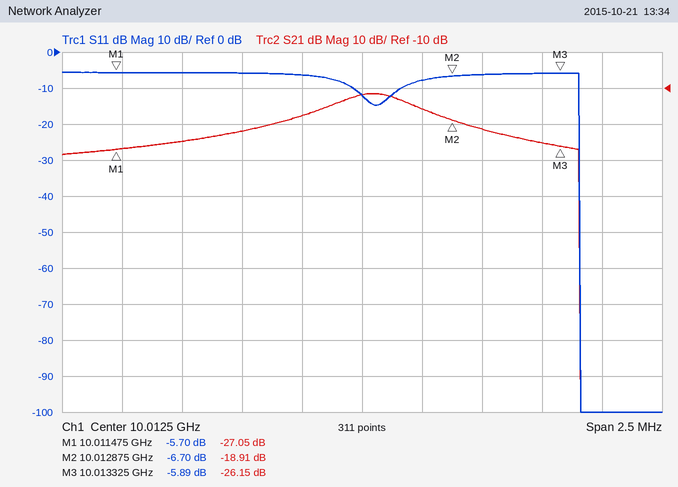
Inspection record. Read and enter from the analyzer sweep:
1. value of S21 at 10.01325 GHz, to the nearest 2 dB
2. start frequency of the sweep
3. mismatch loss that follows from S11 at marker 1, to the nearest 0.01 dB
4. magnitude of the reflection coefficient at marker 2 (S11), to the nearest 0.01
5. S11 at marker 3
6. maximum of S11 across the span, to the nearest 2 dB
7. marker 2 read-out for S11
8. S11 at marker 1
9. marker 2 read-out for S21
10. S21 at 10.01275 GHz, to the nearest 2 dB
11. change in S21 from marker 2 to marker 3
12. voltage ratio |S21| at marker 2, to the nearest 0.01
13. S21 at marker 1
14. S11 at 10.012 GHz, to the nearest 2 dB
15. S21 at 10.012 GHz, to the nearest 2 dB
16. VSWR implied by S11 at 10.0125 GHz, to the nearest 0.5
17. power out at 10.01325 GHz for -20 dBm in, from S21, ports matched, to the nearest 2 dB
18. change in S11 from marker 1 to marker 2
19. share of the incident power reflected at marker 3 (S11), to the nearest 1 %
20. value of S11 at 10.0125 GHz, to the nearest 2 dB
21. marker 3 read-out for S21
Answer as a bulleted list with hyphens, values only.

- -26 dB
- 10.01125 GHz
- 1.36 dB
- 0.46
- -5.89 dB
- -6 dB
- -6.70 dB
- -5.70 dB
- -18.91 dB
- -16 dB
- -7.24 dB
- 0.11
- -27.05 dB
- -6 dB
- -22 dB
- 1.5
- -46 dBm
- -1.00 dB
- 26 %
- -12 dB
- -26.15 dB
